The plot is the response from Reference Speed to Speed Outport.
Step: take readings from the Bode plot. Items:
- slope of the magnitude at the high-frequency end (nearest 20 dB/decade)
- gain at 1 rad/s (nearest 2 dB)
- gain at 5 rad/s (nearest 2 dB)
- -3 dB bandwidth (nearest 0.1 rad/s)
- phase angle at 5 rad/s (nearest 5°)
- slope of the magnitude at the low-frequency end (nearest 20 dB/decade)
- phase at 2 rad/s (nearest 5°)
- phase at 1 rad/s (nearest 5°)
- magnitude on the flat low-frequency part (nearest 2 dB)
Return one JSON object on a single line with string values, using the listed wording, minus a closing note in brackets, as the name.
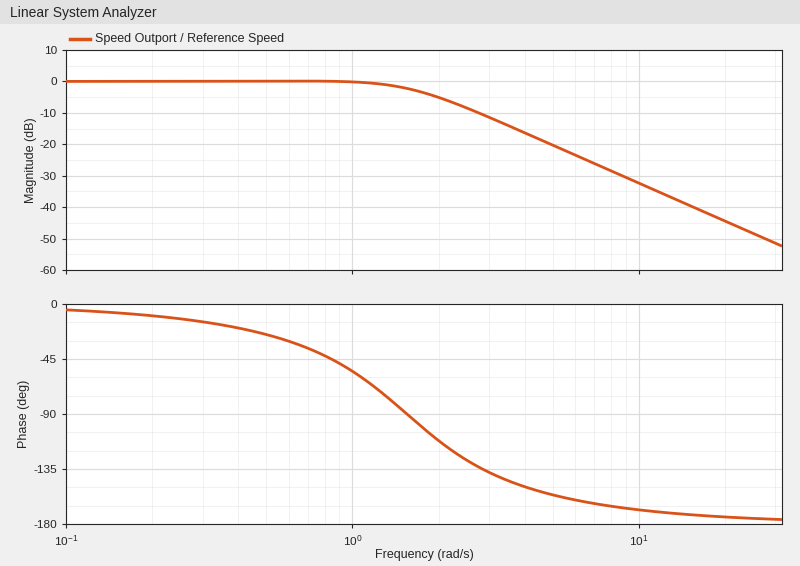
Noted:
{"slope of the magnitude at the high-frequency end": "-40 dB/decade", "gain at 1 rad/s": "0 dB", "gain at 5 rad/s": "-20 dB", "-3 dB bandwidth": "1.7 rad/s", "phase angle at 5 rad/s": "-155°", "slope of the magnitude at the low-frequency end": "0 dB/decade", "phase at 2 rad/s": "-110°", "phase at 1 rad/s": "-55°", "magnitude on the flat low-frequency part": "0 dB"}
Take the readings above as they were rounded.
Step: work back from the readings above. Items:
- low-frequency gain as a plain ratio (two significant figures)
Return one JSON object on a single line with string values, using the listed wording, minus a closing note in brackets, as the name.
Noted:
{"low-frequency gain as a plain ratio": "1.0"}
